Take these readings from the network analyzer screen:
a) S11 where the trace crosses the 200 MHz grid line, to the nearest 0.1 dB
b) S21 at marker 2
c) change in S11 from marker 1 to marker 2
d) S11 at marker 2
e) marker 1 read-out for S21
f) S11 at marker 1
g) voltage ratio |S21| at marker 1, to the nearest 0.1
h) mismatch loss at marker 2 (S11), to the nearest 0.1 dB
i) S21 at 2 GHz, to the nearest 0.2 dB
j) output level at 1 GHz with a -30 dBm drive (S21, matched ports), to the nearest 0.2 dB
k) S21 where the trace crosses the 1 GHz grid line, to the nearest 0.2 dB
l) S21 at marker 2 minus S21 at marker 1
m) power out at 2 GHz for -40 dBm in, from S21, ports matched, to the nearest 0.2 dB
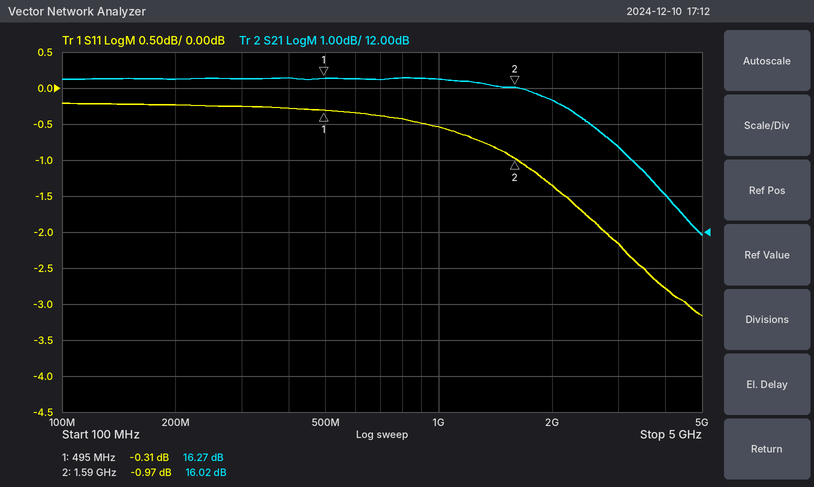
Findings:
-0.2 dB
16.02 dB
-0.66 dB
-0.97 dB
16.27 dB
-0.31 dB
6.5
7.0 dB
15.6 dB
-13.8 dBm
16.2 dB
-0.25 dB
-24.4 dBm
